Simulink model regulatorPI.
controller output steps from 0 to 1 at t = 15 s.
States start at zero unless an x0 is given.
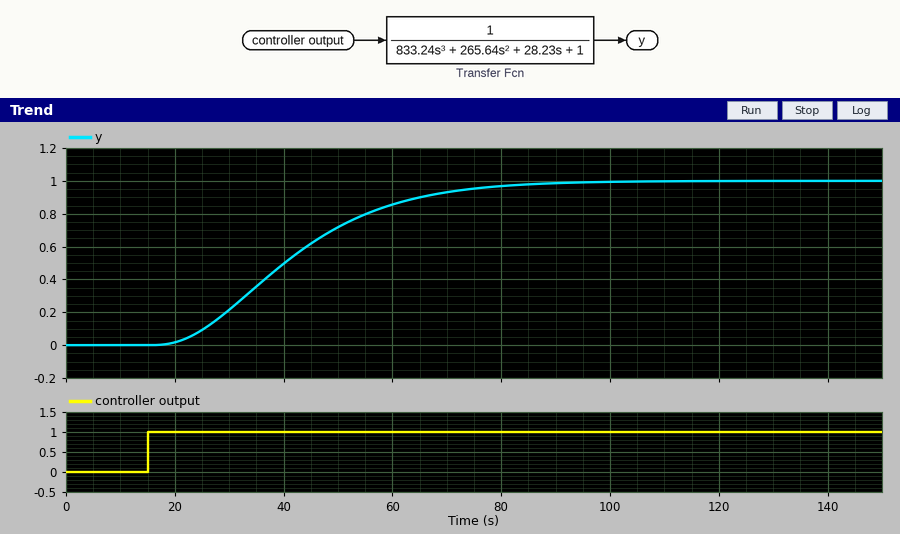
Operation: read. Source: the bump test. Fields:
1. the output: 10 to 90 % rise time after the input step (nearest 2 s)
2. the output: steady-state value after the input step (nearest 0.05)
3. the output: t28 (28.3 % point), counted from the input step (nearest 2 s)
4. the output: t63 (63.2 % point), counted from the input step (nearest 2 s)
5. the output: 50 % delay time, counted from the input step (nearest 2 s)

40 s
1.00
18 s
30 s
26 s
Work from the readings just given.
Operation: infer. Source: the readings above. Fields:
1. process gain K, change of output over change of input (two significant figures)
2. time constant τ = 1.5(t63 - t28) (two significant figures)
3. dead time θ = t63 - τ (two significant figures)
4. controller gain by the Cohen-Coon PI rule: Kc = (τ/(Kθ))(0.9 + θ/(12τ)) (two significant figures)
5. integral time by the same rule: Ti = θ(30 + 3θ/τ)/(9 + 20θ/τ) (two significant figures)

1.0
18 s
12 s
1.4
17 s
